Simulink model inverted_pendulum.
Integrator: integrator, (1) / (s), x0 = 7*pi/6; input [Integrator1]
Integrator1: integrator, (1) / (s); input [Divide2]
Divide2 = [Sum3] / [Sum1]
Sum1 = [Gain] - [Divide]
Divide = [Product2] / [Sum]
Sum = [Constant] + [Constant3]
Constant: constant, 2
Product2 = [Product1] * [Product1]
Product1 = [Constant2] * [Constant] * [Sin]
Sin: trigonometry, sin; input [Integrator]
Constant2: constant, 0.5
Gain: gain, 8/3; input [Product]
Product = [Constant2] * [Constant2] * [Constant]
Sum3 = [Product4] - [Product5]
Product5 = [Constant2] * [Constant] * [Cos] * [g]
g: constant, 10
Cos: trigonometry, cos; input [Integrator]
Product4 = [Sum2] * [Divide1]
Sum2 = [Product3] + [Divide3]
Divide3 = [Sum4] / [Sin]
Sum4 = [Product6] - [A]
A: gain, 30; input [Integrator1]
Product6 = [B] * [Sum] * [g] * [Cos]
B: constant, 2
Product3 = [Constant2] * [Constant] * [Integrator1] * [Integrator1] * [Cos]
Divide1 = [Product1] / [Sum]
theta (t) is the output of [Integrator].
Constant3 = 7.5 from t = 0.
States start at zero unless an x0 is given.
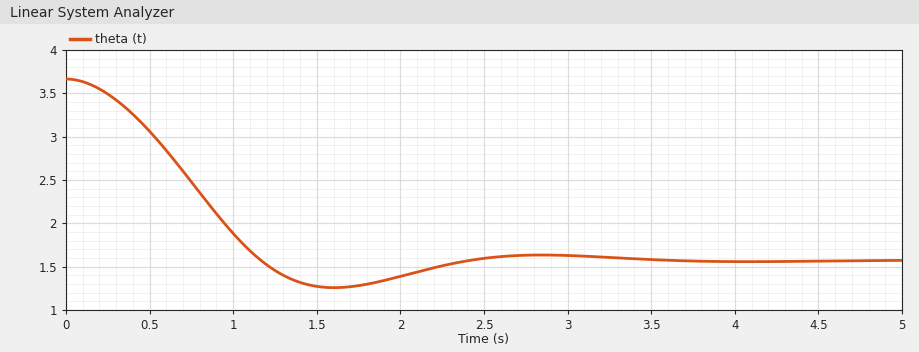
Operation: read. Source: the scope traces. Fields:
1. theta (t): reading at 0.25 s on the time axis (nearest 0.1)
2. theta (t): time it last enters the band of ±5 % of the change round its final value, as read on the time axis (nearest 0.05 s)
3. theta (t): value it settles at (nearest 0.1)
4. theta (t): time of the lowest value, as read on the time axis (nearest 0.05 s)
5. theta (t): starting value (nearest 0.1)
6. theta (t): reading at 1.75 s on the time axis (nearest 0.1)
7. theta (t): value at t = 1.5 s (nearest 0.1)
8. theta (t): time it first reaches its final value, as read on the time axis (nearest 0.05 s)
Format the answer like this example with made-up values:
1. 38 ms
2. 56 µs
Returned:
1. 3.5
2. 2.15 s
3. 1.6
4. 1.60 s
5. 3.7
6. 1.3
7. 1.3
8. 1.15 s
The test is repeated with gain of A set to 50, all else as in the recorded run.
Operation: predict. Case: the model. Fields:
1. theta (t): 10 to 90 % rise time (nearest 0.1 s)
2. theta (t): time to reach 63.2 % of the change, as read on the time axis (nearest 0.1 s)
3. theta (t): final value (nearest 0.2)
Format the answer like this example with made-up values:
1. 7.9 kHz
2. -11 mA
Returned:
1. 1.1 s
2. 1.0 s
3. 1.6
